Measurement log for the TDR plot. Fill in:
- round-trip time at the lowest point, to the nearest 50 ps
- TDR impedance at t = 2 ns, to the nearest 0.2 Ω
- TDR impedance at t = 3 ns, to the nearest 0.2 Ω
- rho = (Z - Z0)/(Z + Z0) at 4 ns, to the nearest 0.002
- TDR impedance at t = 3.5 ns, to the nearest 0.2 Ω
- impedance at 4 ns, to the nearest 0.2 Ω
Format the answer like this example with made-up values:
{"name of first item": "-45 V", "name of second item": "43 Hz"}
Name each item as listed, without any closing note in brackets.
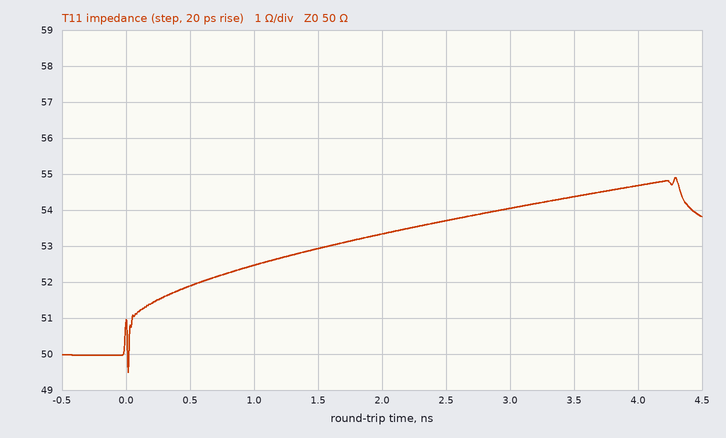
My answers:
{"round-trip time at the lowest point, to the nearest 50 ps": "0 ps", "TDR impedance at t = 2 ns, to the nearest 0.2 Ω": "53.4 Ω", "TDR impedance at t = 3 ns, to the nearest 0.2 Ω": "54.0 Ω", "rho = (Z - Z0)/(Z + Z0) at 4 ns, to the nearest 0.002": "+0.044", "TDR impedance at t = 3.5 ns, to the nearest 0.2 Ω": "54.4 Ω", "impedance at 4 ns, to the nearest 0.2 Ω": "54.6 Ω"}
